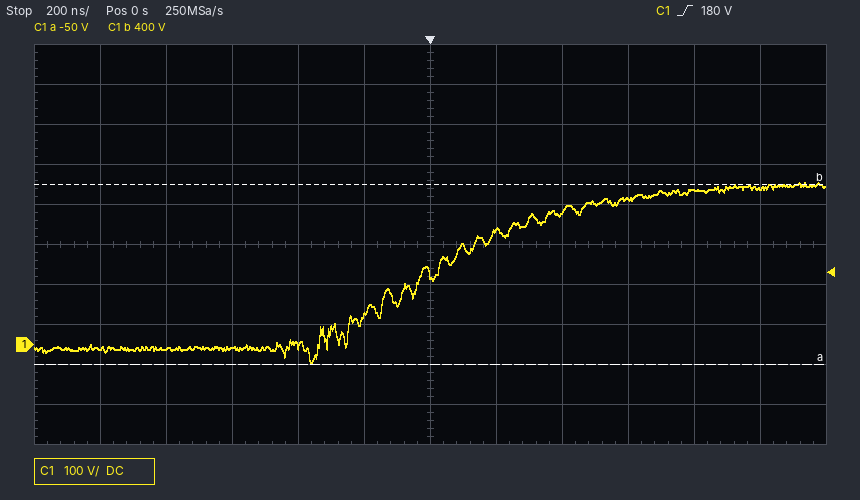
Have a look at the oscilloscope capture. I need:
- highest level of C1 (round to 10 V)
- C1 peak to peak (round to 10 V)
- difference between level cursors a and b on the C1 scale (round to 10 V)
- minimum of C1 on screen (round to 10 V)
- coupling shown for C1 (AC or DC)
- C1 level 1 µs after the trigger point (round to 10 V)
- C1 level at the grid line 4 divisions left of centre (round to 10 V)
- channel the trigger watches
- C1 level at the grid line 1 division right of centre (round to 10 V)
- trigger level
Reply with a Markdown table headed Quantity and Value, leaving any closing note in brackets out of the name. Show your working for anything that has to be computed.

| Quantity | Value |
|---|---|
| highest level of C1 | 400 V |
| C1 peak to peak | 400 V − (-50 V) = 450 V |
| difference between level cursors a and b on the C1 scale | 450 V |
| minimum of C1 on screen | -50 V |
| coupling shown for C1 | DC |
| C1 level 1 µs after the trigger point | 390 V |
| C1 level at the grid line 4 divisions left of centre | -10 V |
| channel the trigger watches | C1 |
| C1 level at the grid line 1 division right of centre | 290 V |
| trigger level | 180 V |
